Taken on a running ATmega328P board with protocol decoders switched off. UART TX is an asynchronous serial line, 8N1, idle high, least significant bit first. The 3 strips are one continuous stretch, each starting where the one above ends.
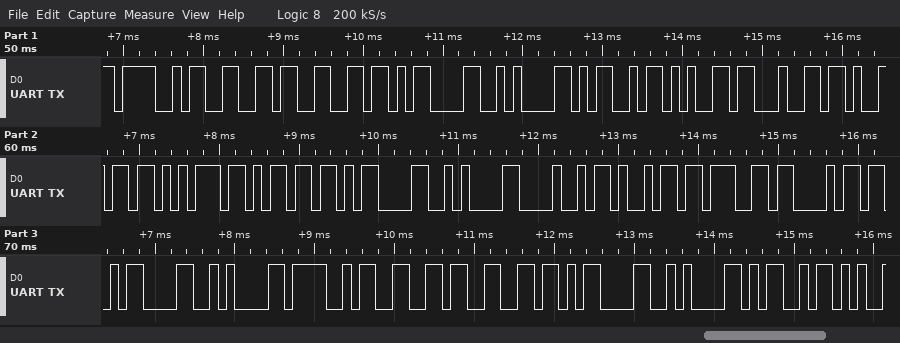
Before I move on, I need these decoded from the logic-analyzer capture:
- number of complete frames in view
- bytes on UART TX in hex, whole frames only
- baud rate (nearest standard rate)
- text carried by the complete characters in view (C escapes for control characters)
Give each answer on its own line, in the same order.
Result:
25
4F 66 66 0D 0A 4D 65 64 69 75 6D 0D 0A 48 69 67 68 0D 0A 4F 66 66 0D 0A 4D
9600 baud
"Off\r\nMedium\r\nHigh\r\nOff\r\nM"
